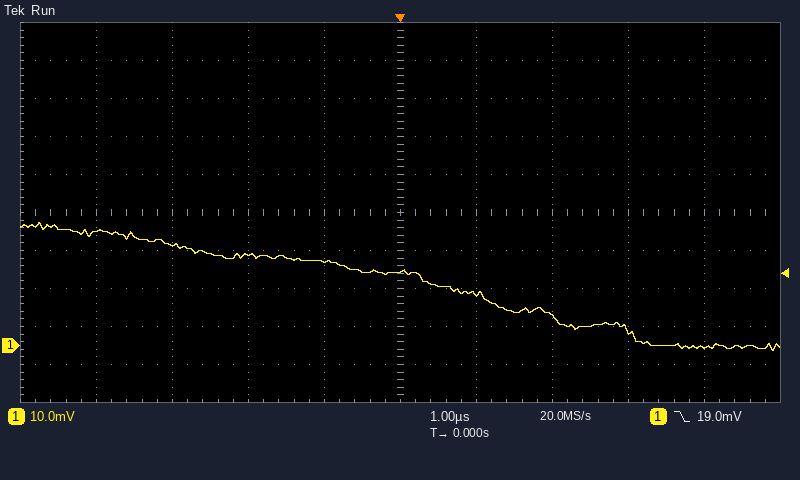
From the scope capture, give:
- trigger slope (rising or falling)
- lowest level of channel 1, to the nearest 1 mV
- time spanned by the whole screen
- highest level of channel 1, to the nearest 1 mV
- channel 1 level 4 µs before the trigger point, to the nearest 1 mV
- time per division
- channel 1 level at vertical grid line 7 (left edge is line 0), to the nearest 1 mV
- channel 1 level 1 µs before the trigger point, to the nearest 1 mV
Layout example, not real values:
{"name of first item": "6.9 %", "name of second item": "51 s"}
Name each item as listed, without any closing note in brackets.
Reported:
{"trigger slope": "falling", "lowest level of channel 1, to the nearest 1 mV": "-1 mV", "time spanned by the whole screen": "10 µs", "highest level of channel 1, to the nearest 1 mV": "32 mV", "channel 1 level 4 µs before the trigger point, to the nearest 1 mV": "30 mV", "time per division": "1 µs", "channel 1 level at vertical grid line 7 (left edge is line 0), to the nearest 1 mV": "8 mV", "channel 1 level 1 µs before the trigger point, to the nearest 1 mV": "22 mV"}
